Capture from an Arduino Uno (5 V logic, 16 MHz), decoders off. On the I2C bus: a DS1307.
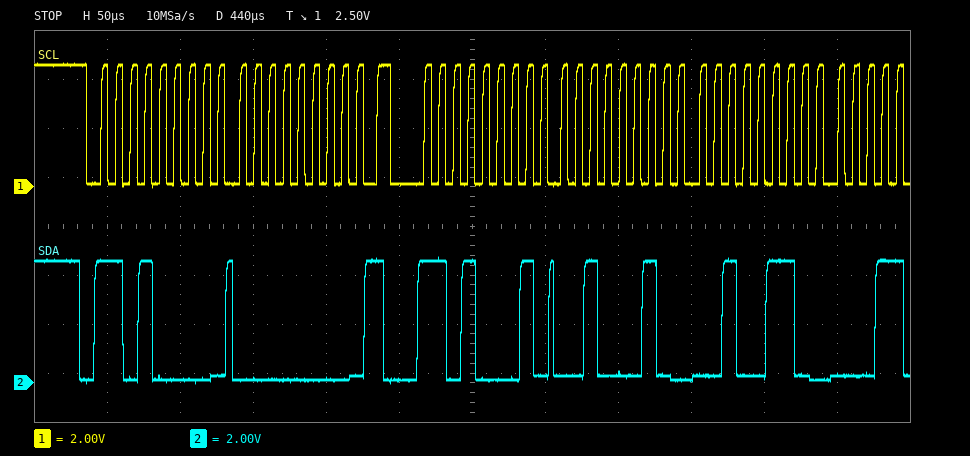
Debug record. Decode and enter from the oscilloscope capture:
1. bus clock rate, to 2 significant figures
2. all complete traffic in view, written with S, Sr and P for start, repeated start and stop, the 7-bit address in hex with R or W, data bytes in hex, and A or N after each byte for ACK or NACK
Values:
100 kHz
S 68W A 00 A Sr 68R A 22 A 26 A
